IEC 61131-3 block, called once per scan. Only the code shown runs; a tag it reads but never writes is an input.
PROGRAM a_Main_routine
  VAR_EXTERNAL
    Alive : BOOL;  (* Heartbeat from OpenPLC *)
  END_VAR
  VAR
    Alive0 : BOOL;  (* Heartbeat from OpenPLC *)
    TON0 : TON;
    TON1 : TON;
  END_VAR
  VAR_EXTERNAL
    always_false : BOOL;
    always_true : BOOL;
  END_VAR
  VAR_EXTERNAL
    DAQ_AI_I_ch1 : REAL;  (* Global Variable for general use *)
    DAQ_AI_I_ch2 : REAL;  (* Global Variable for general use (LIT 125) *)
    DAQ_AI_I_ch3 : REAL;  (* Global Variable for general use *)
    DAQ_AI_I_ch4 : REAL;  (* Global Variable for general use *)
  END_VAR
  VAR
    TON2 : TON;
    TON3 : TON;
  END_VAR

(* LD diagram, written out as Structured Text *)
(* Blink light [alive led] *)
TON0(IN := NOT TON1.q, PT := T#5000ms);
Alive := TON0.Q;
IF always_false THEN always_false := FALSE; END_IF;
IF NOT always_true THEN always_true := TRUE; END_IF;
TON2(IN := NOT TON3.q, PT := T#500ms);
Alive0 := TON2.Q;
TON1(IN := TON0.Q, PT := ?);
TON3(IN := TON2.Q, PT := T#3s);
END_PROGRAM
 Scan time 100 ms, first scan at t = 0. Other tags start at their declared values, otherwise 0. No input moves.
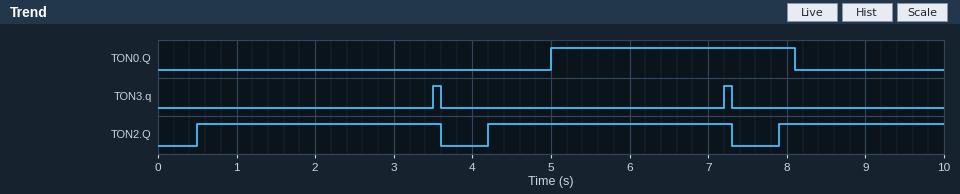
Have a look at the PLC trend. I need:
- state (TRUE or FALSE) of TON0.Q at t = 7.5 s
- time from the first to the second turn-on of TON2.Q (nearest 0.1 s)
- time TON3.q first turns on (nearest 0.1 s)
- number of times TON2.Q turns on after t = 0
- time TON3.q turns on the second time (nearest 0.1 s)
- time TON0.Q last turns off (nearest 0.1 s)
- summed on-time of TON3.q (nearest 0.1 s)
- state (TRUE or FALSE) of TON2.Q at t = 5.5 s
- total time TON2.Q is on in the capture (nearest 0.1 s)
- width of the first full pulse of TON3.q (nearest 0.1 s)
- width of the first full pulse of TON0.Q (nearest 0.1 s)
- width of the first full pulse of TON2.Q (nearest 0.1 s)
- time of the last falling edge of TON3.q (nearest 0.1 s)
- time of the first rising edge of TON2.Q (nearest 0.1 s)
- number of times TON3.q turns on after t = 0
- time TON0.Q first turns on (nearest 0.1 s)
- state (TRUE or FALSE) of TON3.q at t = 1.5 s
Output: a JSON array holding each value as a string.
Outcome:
["TRUE", "3.7 s", "3.5 s", "3", "7.2 s", "8.1 s", "0.2 s", "TRUE", "8.3 s", "0.1 s", "3.1 s", "3.1 s", "7.3 s", "0.5 s", "2", "5.0 s", "FALSE"]
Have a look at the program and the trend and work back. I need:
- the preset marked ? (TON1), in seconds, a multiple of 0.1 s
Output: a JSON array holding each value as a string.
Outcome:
["3.0 s"]
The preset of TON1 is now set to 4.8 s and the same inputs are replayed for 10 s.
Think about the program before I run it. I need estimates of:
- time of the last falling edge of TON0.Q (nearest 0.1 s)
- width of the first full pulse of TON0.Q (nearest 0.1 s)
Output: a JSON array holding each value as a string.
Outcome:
["9.9 s", "4.9 s"]
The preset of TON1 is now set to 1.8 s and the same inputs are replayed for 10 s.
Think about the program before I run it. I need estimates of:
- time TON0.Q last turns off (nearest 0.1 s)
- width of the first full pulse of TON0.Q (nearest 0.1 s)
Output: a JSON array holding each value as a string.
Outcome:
["6.9 s", "1.9 s"]
